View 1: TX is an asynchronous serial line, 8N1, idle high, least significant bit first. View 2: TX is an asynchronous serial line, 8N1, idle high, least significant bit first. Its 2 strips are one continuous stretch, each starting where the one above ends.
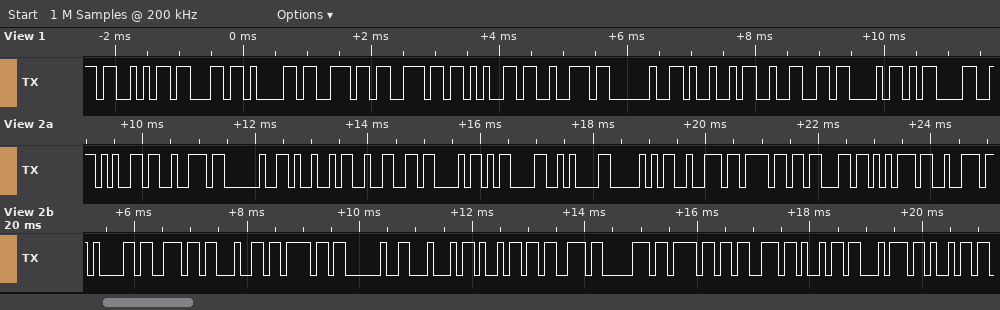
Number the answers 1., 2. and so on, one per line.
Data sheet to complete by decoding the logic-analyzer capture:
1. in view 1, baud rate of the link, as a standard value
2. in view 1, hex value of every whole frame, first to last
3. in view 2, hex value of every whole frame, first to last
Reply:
1. 9600 baud
2. 53 63 61 6E 6E 65 72 20 49 32 43 0D
3. 0x65 0x72 0x20 0x49 0x32 0x43 0x0D 0x0A 0x50 0x72 0x6F 0x63 0x75 0x72 0x61 0x6E 0x64 0x6F 0x20 0x44 0x69 0x73 0x70 0x6F 0x73 0x69 0x74 0x69
